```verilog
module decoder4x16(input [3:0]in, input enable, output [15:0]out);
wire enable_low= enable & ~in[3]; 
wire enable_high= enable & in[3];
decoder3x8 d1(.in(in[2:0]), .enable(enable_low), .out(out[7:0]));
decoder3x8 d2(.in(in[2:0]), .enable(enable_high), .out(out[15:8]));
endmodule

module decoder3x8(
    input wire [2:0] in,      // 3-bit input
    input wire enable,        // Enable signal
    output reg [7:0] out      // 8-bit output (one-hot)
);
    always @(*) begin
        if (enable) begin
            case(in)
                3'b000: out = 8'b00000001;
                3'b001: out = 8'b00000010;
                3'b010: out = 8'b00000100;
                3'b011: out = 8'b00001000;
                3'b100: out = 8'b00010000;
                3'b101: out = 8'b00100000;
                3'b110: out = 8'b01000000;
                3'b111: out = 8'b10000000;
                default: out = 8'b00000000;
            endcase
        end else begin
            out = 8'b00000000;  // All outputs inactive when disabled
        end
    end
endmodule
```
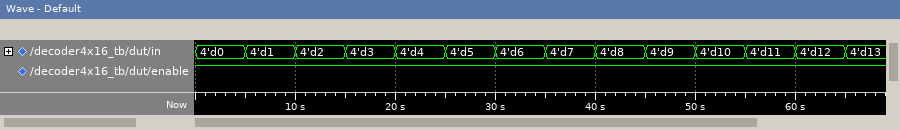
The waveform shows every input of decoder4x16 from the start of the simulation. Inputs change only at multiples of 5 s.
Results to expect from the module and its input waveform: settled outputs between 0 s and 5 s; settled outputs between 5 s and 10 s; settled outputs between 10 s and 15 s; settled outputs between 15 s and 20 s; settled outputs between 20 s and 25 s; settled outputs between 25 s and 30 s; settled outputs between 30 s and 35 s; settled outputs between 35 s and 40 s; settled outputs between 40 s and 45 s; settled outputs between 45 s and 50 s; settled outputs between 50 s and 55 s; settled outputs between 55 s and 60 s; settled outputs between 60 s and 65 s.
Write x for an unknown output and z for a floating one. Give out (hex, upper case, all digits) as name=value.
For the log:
out=0001
out=0002
out=0004
out=0008
out=0010
out=0020
out=0040
out=0080
out=0100
out=0200
out=0400
out=0800
out=1000
